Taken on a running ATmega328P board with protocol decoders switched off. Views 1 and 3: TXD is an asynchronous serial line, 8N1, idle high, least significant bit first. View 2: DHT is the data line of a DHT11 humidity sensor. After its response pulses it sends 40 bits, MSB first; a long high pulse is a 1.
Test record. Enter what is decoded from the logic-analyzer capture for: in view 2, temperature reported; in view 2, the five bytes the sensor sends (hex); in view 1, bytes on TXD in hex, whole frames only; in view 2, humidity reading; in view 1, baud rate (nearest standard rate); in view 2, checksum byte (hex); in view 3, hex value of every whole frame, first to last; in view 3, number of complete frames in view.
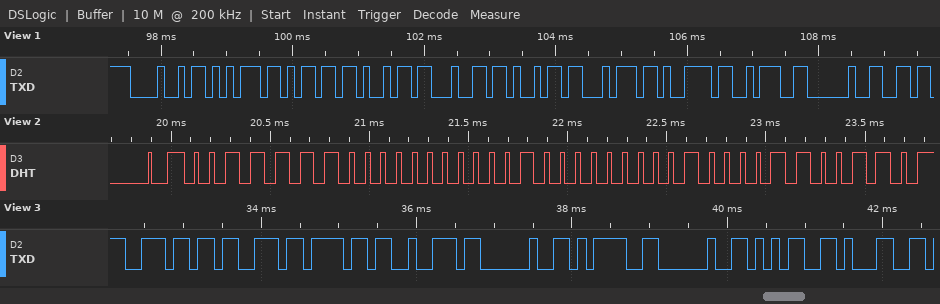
32.8 °C
3E 00 20 08 66
0x48 0x75 0x6D 0x69 0x64 0x69 0x74 0x79 0x3A 0x20
62 %
9600 baud
0x66
6E 73 6F 72 20 3D 20 35 31
9
